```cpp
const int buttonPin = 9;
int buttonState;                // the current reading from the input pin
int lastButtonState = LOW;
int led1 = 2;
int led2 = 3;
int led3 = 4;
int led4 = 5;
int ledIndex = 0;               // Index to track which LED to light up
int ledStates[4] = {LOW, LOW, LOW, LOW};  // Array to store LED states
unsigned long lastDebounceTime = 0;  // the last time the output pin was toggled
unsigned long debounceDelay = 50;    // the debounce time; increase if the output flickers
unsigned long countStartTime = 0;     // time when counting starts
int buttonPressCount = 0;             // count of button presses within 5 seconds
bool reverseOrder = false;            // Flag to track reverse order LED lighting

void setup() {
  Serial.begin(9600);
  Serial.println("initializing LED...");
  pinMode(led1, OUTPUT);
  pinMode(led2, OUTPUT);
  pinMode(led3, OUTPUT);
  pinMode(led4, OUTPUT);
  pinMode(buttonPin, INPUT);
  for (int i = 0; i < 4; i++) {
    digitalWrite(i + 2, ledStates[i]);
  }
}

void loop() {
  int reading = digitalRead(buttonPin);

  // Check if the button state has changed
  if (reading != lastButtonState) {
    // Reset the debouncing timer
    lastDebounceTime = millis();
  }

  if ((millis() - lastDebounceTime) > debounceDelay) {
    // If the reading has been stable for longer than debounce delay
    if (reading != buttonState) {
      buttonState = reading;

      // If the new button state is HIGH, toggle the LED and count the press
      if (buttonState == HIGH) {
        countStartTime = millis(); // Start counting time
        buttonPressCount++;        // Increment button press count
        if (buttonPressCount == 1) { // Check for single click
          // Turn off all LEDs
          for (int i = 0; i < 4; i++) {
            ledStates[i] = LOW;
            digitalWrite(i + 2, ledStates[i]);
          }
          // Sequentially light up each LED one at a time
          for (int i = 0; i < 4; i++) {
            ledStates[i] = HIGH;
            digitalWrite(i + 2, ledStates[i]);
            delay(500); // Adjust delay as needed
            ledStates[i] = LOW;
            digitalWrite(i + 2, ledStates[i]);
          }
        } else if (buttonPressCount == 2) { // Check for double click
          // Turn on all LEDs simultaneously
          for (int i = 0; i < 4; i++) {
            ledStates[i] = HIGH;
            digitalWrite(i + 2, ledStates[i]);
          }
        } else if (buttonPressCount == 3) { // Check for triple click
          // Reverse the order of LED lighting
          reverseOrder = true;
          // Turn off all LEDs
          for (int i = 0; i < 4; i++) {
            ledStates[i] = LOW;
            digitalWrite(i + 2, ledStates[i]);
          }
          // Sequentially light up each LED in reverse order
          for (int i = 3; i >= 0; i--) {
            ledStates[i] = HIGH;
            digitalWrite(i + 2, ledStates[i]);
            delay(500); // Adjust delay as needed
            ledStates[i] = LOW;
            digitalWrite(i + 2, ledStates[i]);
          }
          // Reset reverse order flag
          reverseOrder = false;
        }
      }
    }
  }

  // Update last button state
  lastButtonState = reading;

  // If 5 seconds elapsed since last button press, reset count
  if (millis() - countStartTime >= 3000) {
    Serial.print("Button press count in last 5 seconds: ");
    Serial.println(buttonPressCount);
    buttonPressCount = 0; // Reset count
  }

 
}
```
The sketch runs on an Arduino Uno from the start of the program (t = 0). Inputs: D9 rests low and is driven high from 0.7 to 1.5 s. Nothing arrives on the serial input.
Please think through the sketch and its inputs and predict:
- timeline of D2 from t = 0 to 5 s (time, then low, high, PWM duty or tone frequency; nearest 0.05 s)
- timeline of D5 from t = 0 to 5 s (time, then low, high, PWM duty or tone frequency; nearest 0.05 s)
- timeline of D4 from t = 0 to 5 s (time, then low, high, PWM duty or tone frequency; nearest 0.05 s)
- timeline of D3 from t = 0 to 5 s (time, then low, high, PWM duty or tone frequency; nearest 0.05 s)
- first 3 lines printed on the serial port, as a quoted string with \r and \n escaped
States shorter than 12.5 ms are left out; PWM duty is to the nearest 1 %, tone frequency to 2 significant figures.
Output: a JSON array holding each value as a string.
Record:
["0 s low; 0.75 s high; 1.25 s low", "0 s low; 2.25 s high; 2.75 s low", "0 s low; 1.75 s high; 2.25 s low", "0 s low; 1.25 s high; 1.75 s low", "\"initializing LED...\\r\\nButton press count in last 5 seconds: 1\\r\\nButton press count in last 5 seconds: 0\\r\\n\""]
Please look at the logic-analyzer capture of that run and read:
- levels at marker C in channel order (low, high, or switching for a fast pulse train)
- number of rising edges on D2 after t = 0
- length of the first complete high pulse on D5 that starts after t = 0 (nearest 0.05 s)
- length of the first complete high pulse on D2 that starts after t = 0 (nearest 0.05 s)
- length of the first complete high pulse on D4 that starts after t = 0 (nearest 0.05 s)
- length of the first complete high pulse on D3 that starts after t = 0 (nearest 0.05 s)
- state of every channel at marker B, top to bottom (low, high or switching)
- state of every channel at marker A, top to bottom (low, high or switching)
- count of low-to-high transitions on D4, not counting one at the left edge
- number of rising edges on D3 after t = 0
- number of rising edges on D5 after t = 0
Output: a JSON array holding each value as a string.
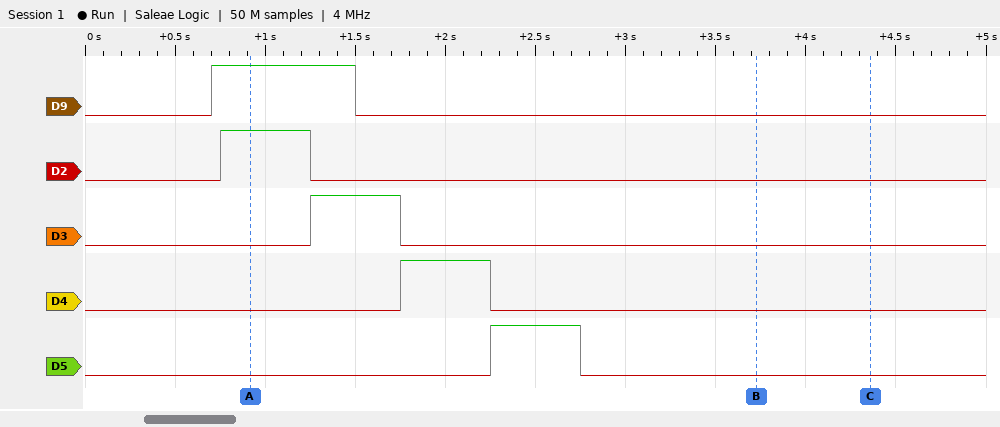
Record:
["D9 low, D2 low, D3 low, D4 low, D5 low", "1", "0.50 s", "0.50 s", "0.50 s", "0.50 s", "D9 low, D2 low, D3 low, D4 low, D5 low", "D9 high, D2 high, D3 low, D4 low, D5 low", "1", "1", "1"]
